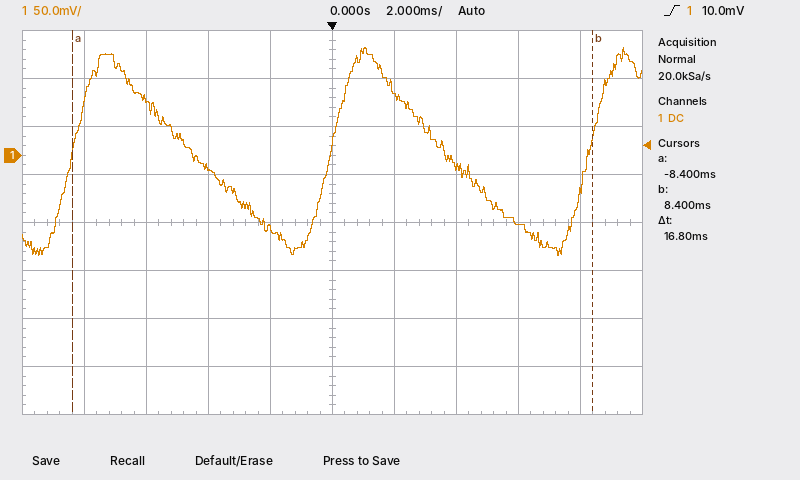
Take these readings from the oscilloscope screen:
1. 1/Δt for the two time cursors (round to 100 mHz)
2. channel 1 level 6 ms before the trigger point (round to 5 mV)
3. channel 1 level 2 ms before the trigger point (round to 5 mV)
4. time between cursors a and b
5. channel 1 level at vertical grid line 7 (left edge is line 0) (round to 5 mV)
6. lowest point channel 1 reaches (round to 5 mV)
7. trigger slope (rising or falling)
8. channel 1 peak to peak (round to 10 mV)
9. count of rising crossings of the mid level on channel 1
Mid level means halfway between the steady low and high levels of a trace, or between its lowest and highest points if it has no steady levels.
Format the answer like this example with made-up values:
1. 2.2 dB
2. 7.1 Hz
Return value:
1. 59.5 Hz
2. 60 mV
3. -75 mV
4. 16.8 ms
5. -10 mV
6. -105 mV
7. rising
8. 220 mV
9. 3
